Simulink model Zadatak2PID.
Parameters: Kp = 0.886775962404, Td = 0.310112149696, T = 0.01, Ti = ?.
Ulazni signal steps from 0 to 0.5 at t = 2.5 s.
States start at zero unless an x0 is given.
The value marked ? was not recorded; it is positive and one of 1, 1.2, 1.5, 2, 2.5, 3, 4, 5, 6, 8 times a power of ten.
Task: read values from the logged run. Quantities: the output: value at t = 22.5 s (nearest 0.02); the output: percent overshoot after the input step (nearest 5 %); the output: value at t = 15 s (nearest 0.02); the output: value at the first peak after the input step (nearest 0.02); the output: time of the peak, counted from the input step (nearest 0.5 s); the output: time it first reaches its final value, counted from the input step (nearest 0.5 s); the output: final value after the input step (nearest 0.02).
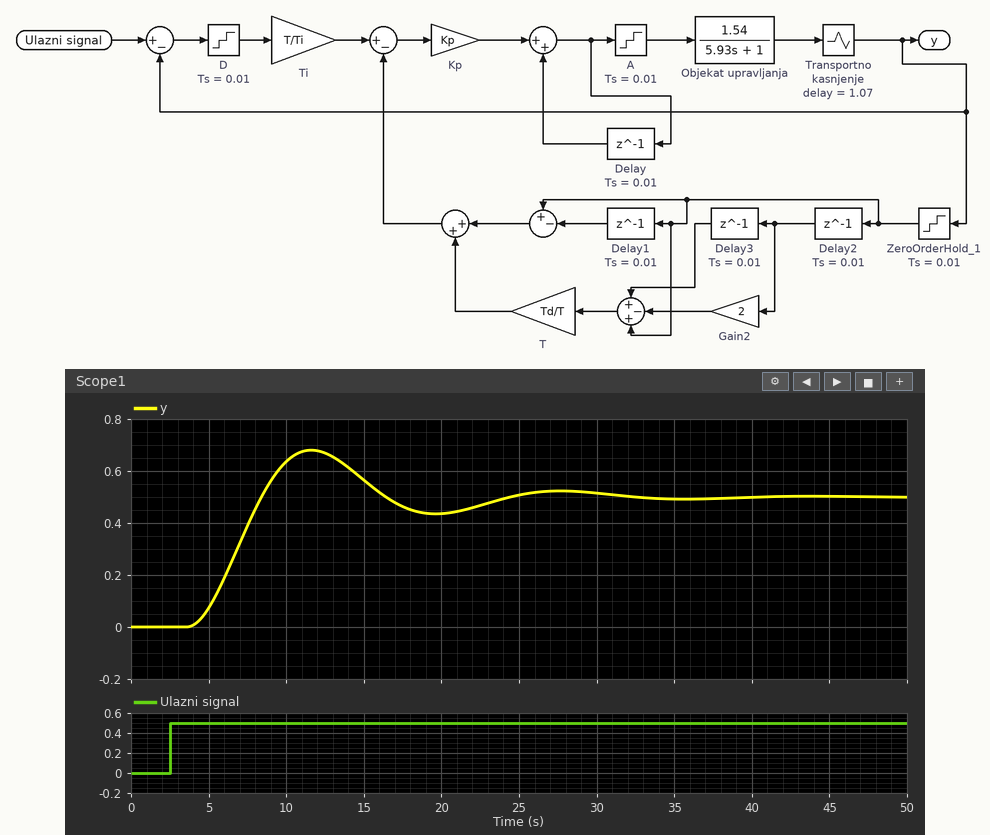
0.46
35 %
0.56
0.68
9.0 s
6.0 s
0.50
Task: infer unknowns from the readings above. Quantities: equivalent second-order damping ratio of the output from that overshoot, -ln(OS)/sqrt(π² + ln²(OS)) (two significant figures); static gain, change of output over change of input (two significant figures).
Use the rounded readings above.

0.32
1.0
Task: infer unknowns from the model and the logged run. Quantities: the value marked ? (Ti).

1.5
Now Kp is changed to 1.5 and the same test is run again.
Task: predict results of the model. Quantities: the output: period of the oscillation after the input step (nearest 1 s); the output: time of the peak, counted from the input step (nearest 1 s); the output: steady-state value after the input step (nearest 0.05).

12 s
7 s
0.50
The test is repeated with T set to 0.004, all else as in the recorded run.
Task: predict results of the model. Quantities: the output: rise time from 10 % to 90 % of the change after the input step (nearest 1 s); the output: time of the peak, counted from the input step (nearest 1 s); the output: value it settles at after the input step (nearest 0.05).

8 s
18 s
0.50
